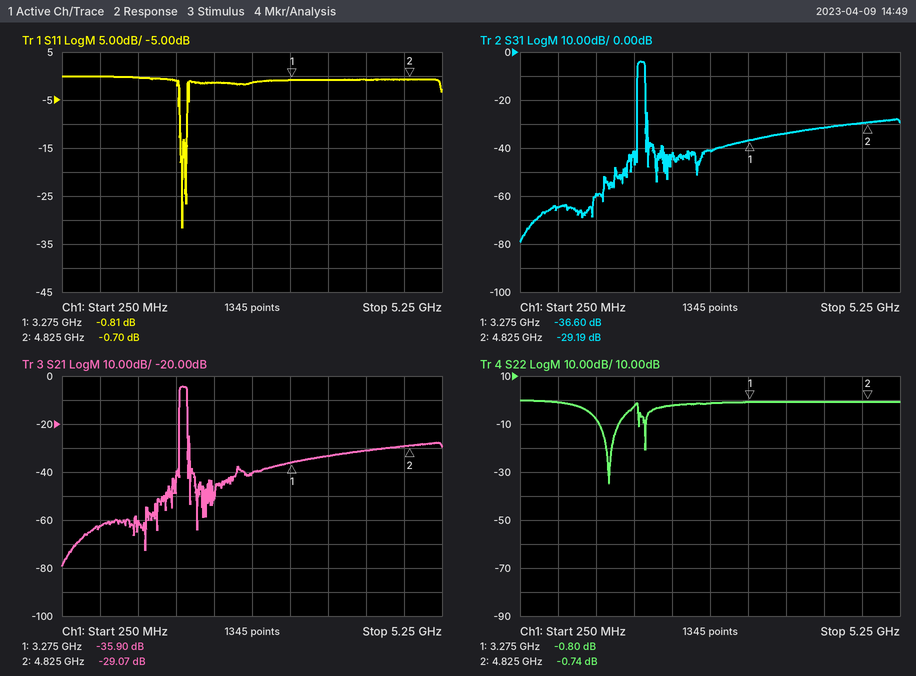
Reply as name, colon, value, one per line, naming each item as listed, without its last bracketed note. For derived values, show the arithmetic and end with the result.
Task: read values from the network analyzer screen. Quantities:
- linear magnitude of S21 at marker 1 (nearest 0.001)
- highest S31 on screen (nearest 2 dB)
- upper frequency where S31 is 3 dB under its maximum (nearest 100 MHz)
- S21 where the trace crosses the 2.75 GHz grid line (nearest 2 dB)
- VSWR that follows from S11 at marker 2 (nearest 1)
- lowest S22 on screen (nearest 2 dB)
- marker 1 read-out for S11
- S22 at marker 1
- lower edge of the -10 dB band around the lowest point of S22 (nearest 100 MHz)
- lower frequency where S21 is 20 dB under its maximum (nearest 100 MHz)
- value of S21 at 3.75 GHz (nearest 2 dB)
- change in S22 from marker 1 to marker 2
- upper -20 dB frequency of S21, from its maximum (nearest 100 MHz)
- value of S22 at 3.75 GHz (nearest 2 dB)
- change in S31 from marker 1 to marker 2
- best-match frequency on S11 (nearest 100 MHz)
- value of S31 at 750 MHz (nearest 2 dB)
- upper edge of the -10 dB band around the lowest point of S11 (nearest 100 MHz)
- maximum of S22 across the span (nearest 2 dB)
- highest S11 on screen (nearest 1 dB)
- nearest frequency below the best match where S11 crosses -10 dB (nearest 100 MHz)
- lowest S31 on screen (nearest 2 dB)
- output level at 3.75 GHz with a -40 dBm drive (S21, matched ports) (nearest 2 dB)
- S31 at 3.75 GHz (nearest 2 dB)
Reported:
linear magnitude of S21 at marker 1: 10^(-35.9/20) ≈ 0.016
highest S31 on screen: -4 dB
upper frequency where S31 is 3 dB under its maximum: 1.9 GHz
S21 where the trace crosses the 2.75 GHz grid line: -40 dB
VSWR that follows from S11 at marker 2: (1 + 0.9226)/(1 − 0.9226) ≈ 25
lowest S22 on screen: -34 dB
marker 1 read-out for S11: -0.81 dB
S22 at marker 1: -0.80 dB
lower edge of the -10 dB band around the lowest point of S22: 1.3 GHz
lower frequency where S21 is 20 dB under its maximum: 1.8 GHz
value of S21 at 3.75 GHz: -34 dB
change in S22 from marker 1 to marker 2: -0.74 − (-0.8) = 0.06 dB
upper -20 dB frequency of S21, from its maximum: 1.9 GHz
value of S22 at 3.75 GHz: 0 dB
change in S31 from marker 1 to marker 2: -29.19 − (-36.6) = 7.41 dB
best-match frequency on S11: 1.8 GHz
value of S31 at 750 MHz: -64 dB
upper edge of the -10 dB band around the lowest point of S11: 1.9 GHz
maximum of S22 across the span: 0 dB
highest S11 on screen: 0 dB
nearest frequency below the best match where S11 crosses -10 dB: 1.8 GHz
lowest S31 on screen: -80 dB
output level at 3.75 GHz with a -40 dBm drive (S21, matched ports): -40 dBm + (-34 dB) = -74 dBm
S31 at 3.75 GHz: -34 dB
